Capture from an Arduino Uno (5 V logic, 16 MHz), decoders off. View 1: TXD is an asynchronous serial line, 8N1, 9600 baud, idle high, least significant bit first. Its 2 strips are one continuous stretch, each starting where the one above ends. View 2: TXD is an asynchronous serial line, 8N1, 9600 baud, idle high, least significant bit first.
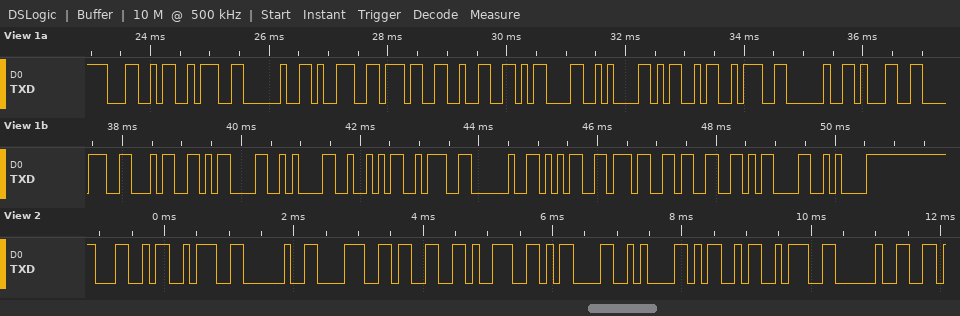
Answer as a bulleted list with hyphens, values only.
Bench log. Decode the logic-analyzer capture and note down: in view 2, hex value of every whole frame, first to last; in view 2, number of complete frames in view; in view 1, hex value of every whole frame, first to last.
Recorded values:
- 4C 3A 20 38 33 39 0D 0A 4D 3A 20
- 11
- 4C 3A 20 39 37 32 0D 0A 4D 3A 20 31 38 34 0D 0A 52 3A 20 35 37 33 0D 0A
